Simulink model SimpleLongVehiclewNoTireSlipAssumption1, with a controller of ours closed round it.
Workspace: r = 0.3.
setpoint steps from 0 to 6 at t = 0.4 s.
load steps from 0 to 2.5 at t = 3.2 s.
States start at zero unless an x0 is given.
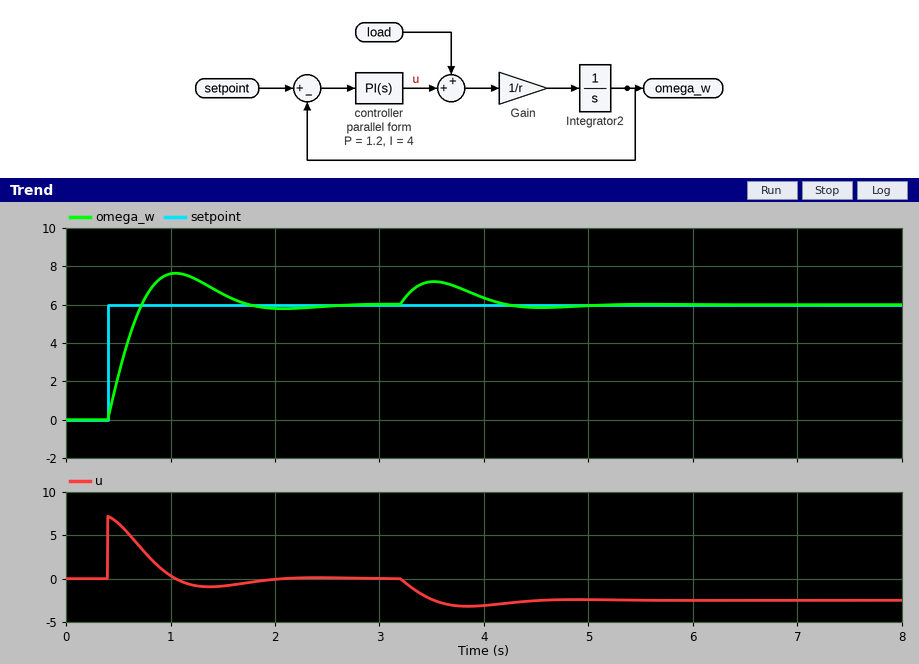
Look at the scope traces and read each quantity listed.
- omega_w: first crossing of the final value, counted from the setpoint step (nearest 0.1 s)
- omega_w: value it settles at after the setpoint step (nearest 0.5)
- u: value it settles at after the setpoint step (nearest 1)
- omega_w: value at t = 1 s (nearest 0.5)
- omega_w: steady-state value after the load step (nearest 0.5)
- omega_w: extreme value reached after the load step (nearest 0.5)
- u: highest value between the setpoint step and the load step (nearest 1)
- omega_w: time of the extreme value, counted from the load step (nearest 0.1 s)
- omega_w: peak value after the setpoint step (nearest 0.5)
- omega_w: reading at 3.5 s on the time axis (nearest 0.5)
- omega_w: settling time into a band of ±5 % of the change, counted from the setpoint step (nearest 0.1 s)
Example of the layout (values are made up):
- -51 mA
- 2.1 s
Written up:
- 0.3 s
- 6.0
- 0
- 7.5
- 6.0
- 7.0
- 7
- 0.3 s
- 7.5
- 7.0
- 1.2 s
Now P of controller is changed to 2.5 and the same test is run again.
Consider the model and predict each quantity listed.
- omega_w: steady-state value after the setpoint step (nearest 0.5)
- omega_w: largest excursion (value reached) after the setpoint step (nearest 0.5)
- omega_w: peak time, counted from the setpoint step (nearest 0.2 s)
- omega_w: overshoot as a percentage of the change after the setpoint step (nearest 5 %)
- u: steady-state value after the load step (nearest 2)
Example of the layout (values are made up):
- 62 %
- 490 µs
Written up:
- 6.0
- 6.5
- 0.6 s
- 10 %
- -2
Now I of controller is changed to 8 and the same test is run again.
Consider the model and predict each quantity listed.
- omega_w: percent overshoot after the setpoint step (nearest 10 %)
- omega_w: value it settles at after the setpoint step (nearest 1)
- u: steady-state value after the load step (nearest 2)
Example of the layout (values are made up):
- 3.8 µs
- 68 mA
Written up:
- 40 %
- 6
- -2
